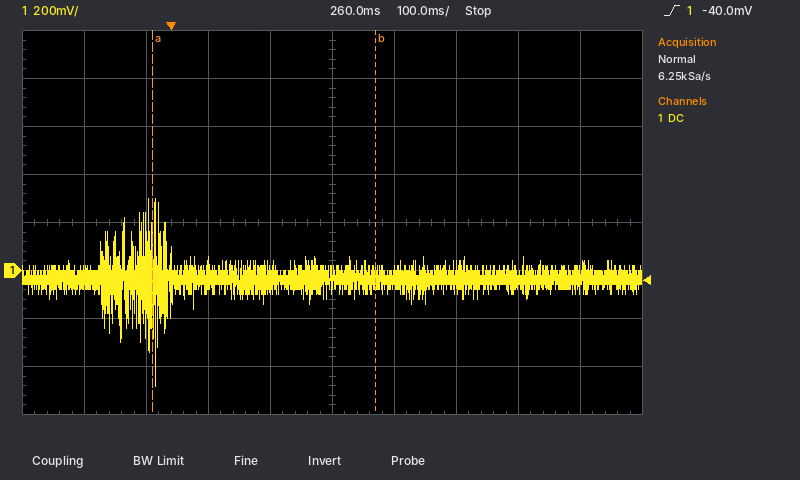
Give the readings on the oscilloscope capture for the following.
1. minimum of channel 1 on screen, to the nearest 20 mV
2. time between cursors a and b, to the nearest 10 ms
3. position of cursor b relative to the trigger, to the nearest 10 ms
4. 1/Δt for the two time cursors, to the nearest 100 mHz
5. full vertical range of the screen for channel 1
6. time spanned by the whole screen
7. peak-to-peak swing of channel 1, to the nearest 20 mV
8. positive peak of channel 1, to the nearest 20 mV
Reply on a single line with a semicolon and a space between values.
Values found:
-480 mV; 360 ms; +330 ms; 2.8 Hz; 1.6 V; 1 s; 780 mV; 300 mV
